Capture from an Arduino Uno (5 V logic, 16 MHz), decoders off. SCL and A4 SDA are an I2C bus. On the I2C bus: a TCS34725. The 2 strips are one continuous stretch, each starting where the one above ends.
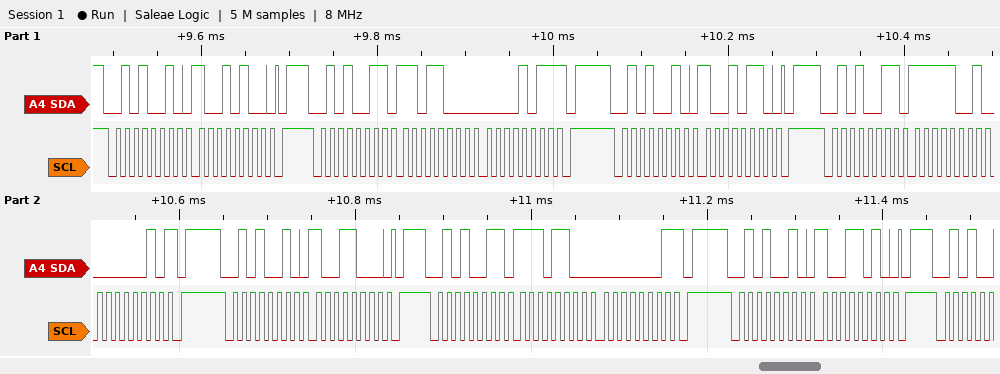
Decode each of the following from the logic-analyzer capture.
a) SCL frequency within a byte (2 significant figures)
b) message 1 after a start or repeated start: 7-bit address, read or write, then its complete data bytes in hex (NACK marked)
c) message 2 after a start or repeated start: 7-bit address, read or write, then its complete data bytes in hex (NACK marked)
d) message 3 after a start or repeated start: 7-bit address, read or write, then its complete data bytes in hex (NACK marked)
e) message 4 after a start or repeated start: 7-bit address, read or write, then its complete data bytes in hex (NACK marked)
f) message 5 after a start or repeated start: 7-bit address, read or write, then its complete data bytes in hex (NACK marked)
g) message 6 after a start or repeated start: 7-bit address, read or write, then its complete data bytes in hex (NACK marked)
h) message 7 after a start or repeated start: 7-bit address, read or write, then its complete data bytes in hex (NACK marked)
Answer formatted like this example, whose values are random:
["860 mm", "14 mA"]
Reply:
["100 kHz", "0x29 write: 94", "0x29 read: D8 0B NACK", "0x29 write: 96", "0x29 read: F9 02 NACK", "0x29 write: 98", "0x29 read: EC 01 NACK", "0x29 write: 9A"]
